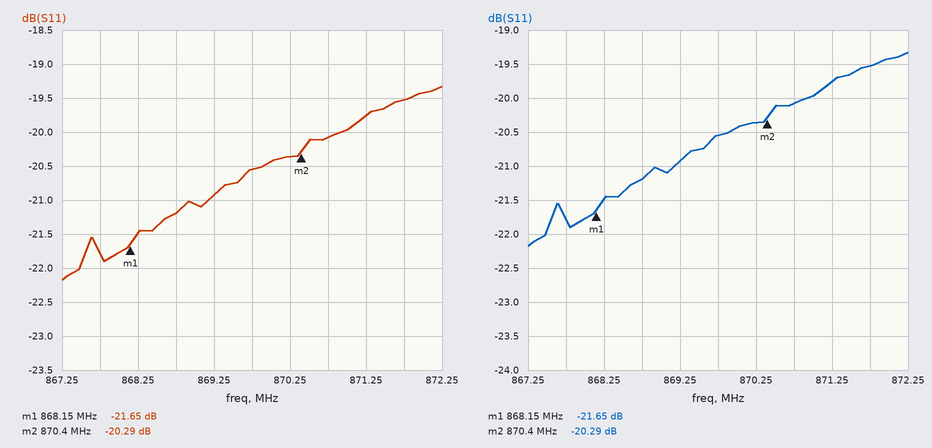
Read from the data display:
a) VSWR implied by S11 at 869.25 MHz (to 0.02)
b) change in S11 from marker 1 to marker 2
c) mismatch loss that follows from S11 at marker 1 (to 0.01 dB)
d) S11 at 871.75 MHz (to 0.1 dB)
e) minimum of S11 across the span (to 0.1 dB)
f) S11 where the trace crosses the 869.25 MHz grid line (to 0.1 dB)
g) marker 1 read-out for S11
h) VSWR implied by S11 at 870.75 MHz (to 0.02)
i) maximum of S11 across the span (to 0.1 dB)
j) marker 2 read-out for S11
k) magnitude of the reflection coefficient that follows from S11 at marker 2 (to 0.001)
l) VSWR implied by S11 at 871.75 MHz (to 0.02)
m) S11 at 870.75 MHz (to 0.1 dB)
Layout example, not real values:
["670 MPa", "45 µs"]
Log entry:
["1.20", "1.36 dB", "0.03 dB", "-19.5 dB", "-22.2 dB", "-20.9 dB", "-21.65 dB", "1.22", "-19.3 dB", "-20.29 dB", "0.097", "1.24", "-20.1 dB"]
